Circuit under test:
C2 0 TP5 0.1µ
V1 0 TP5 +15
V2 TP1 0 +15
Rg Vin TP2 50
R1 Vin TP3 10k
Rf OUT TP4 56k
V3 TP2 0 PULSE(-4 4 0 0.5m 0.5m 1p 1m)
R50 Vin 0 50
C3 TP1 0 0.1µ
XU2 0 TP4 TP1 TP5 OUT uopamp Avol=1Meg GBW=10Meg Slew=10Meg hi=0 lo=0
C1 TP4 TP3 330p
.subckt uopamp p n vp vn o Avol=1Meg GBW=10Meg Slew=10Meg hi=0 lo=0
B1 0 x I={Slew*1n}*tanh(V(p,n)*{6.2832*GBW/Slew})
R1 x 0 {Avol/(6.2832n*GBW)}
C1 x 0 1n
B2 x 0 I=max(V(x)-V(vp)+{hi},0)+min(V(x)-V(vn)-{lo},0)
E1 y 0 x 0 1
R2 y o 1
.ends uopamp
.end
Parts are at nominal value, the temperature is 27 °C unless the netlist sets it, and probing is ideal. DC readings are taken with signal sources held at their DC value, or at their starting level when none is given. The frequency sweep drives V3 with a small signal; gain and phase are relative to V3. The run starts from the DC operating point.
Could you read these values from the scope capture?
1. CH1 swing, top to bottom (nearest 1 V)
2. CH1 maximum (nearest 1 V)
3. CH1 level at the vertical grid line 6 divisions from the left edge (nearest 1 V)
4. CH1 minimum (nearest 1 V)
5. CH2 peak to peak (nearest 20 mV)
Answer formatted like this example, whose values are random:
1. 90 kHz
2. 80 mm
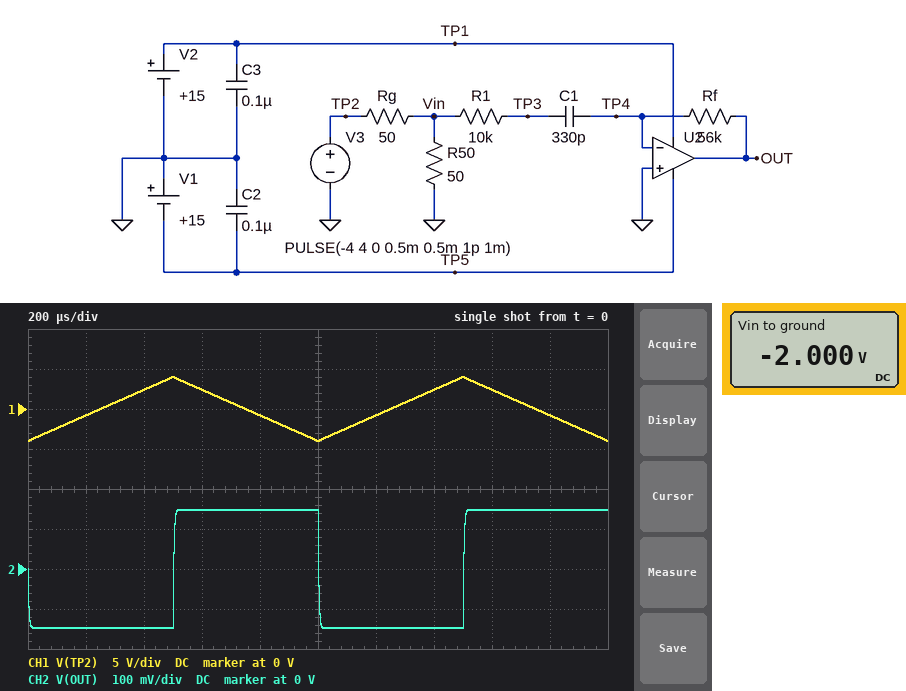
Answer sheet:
1. 8 V
2. 4 V
3. -1 V
4. -4 V
5. 300 mV
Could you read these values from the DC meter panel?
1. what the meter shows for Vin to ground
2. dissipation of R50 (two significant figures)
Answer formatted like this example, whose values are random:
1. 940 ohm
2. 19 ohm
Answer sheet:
1. -2.000 V
2. 80 mW
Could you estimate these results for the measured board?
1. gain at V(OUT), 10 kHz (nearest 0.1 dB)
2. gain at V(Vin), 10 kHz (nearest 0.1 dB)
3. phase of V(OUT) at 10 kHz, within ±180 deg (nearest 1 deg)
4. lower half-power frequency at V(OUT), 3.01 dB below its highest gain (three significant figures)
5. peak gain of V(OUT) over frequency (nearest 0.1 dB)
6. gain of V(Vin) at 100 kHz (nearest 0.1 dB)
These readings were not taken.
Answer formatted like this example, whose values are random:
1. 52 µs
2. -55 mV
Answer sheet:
1. -4.9 dB
2. -6.0 dB
3. -102 deg
4. 46.5 kHz
5. 8.9 dB
6. -6.0 dB
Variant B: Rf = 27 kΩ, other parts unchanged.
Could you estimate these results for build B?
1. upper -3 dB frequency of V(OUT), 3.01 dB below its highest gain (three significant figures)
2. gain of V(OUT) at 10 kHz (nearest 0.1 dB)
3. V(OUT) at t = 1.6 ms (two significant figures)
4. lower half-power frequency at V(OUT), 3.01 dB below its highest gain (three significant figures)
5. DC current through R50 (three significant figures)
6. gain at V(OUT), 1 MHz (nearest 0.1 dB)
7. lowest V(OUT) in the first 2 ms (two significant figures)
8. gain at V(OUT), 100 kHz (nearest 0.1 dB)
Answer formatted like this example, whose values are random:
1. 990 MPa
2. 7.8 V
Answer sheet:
1. 2.77 MHz
2. -11.2 dB
3. 71 mV
4. 47.1 kHz
5. 40.0 mA
6. 2.1 dB
7. -71 mV
8. 1.8 dB
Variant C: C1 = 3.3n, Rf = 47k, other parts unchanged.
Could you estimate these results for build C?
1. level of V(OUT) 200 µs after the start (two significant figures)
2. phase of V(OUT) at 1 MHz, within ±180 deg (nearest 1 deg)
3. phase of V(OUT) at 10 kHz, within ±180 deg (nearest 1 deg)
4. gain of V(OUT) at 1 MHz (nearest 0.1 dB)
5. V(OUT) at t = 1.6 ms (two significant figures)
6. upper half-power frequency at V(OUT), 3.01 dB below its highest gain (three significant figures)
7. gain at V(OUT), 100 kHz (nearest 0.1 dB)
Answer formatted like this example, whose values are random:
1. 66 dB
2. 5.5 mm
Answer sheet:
1. -1.2 V
2. 151 deg
3. -155 deg
4. 6.2 dB
5. 1.1 V
6. 1.76 MHz
7. 7.4 dB
